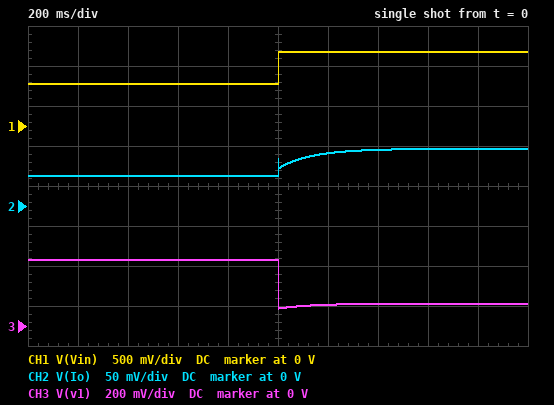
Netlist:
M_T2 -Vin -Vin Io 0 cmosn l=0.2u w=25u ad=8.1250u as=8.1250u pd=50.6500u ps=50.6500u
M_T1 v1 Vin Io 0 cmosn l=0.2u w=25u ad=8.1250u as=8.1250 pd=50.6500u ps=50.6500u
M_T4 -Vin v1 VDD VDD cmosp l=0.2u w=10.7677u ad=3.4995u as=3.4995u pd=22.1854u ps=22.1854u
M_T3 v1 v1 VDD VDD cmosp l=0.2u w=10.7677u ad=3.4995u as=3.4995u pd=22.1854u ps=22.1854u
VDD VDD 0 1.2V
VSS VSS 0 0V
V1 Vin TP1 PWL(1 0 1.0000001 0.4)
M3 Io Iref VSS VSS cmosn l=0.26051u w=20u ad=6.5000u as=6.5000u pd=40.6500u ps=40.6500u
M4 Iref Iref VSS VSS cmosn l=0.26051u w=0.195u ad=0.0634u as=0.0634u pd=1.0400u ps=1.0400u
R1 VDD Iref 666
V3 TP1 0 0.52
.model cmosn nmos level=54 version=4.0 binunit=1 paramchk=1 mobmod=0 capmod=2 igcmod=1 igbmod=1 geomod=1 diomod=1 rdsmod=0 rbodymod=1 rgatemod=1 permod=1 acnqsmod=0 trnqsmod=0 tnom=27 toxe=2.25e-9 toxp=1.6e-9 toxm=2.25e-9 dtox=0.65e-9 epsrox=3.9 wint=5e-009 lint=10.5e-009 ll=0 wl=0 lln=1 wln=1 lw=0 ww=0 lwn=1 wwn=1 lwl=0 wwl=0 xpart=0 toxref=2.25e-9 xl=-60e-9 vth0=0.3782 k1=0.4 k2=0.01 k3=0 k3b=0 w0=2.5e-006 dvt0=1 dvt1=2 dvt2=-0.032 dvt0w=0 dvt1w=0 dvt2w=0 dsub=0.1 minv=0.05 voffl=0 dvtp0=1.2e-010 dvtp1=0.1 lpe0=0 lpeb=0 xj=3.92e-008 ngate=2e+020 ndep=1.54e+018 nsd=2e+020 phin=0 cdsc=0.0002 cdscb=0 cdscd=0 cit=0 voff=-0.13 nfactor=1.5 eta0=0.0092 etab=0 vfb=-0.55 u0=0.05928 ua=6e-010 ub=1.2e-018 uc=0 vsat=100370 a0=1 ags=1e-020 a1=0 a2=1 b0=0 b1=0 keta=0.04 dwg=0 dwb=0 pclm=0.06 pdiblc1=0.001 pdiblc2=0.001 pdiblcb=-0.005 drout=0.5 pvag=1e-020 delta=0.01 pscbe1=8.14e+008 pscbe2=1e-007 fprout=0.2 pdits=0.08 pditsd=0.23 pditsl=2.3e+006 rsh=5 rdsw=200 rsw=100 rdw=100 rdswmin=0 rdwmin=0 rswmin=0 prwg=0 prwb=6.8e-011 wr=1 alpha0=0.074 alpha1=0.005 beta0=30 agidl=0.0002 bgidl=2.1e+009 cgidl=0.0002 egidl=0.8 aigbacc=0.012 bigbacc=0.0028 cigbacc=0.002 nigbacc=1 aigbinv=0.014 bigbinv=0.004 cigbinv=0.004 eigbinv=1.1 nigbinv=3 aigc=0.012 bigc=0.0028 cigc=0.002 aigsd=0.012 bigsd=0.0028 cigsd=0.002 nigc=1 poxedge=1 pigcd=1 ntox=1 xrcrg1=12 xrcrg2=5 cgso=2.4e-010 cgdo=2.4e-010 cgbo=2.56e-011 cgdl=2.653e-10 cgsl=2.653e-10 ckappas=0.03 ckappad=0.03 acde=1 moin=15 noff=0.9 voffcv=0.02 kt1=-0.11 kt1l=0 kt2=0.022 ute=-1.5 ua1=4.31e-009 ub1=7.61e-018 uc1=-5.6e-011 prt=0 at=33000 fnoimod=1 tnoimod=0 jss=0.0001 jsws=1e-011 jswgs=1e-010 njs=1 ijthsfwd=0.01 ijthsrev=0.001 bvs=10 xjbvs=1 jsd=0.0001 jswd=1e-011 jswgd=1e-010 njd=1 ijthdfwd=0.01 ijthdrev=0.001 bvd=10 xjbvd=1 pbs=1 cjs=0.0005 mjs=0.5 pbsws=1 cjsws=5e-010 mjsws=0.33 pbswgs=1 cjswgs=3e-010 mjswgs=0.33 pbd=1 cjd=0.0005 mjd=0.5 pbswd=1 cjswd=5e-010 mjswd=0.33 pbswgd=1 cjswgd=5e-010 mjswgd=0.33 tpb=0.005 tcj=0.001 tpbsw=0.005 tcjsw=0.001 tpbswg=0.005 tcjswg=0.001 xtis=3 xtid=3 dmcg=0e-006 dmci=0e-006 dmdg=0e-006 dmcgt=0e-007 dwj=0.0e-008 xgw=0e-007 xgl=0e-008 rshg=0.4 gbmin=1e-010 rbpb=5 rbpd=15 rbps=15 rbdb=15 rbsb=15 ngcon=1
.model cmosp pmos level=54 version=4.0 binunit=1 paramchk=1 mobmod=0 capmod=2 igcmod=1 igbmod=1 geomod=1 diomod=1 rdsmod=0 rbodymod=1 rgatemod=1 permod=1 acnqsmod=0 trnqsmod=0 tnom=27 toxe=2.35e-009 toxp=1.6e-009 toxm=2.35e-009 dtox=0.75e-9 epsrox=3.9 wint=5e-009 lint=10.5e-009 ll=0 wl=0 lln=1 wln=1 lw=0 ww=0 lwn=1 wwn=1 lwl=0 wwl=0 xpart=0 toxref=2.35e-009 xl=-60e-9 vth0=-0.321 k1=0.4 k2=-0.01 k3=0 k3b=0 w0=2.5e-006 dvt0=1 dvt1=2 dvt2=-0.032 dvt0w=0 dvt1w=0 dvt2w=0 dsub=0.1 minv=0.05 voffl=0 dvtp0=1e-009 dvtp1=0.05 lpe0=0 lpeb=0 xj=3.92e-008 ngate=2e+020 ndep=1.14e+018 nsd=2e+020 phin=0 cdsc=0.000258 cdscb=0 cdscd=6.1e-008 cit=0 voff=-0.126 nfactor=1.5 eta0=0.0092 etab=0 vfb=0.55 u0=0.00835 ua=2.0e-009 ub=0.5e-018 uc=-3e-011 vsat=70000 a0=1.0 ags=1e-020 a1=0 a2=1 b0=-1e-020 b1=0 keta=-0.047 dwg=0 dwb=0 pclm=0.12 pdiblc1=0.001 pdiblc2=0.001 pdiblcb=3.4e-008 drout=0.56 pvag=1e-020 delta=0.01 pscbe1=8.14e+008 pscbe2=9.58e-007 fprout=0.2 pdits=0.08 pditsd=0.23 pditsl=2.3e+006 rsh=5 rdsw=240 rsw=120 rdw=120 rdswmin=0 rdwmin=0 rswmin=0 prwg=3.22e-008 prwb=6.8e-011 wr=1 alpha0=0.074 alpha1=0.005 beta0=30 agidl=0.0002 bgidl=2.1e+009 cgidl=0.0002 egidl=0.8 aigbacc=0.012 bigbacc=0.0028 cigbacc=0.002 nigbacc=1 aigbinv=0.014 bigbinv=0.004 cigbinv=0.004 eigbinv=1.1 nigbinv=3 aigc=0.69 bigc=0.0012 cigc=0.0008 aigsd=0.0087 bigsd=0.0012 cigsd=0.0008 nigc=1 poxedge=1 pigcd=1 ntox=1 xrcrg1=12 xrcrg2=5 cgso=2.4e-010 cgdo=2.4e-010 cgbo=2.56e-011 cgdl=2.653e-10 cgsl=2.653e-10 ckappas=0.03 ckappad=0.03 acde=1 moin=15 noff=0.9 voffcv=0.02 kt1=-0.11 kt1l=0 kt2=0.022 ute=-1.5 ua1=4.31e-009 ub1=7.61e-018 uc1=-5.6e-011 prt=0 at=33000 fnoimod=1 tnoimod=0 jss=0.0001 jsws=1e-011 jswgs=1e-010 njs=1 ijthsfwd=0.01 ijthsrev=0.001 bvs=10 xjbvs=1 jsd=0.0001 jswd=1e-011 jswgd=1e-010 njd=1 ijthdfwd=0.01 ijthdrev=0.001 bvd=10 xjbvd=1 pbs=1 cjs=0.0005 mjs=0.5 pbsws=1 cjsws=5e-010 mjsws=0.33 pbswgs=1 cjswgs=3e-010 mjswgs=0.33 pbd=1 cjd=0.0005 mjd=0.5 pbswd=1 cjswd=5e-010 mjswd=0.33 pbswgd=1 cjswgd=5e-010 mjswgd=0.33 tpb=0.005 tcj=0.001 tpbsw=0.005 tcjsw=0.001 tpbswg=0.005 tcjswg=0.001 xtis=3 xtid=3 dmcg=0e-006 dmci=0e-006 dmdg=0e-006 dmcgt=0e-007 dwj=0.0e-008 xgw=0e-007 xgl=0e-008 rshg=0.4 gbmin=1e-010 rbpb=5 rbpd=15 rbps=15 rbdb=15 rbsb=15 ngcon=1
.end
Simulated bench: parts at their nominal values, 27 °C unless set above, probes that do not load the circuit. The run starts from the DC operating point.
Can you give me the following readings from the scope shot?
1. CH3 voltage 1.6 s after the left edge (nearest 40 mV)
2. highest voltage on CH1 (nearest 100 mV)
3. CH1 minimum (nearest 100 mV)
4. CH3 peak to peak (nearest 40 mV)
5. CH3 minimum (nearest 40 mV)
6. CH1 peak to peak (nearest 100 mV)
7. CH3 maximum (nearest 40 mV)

120 mV
900 mV
500 mV
240 mV
80 mV
400 mV
320 mV
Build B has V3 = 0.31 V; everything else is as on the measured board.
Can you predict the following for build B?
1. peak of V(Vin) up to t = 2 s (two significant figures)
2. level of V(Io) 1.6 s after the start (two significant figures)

710 mV
68 mV
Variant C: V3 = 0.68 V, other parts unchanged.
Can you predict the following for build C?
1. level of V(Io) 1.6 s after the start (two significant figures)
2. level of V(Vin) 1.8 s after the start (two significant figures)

72 mV
1.1 V
